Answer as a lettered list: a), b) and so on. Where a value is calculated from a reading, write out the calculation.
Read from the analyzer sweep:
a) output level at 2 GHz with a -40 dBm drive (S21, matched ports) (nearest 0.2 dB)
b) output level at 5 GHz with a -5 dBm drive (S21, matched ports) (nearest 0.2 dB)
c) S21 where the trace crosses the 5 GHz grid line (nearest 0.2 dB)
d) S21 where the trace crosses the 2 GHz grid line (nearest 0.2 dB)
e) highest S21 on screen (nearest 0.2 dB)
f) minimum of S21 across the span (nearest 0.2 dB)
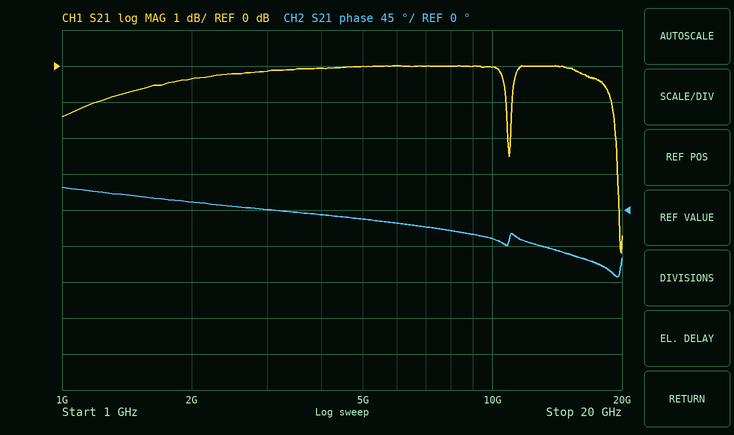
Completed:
a) -40 dBm + (-0.4 dB) = -40.4 dBm
b) -5 dBm + (0.0 dB) = -5.0 dBm
c) 0.0 dB
d) -0.4 dB
e) 0.0 dB
f) -5.2 dB
